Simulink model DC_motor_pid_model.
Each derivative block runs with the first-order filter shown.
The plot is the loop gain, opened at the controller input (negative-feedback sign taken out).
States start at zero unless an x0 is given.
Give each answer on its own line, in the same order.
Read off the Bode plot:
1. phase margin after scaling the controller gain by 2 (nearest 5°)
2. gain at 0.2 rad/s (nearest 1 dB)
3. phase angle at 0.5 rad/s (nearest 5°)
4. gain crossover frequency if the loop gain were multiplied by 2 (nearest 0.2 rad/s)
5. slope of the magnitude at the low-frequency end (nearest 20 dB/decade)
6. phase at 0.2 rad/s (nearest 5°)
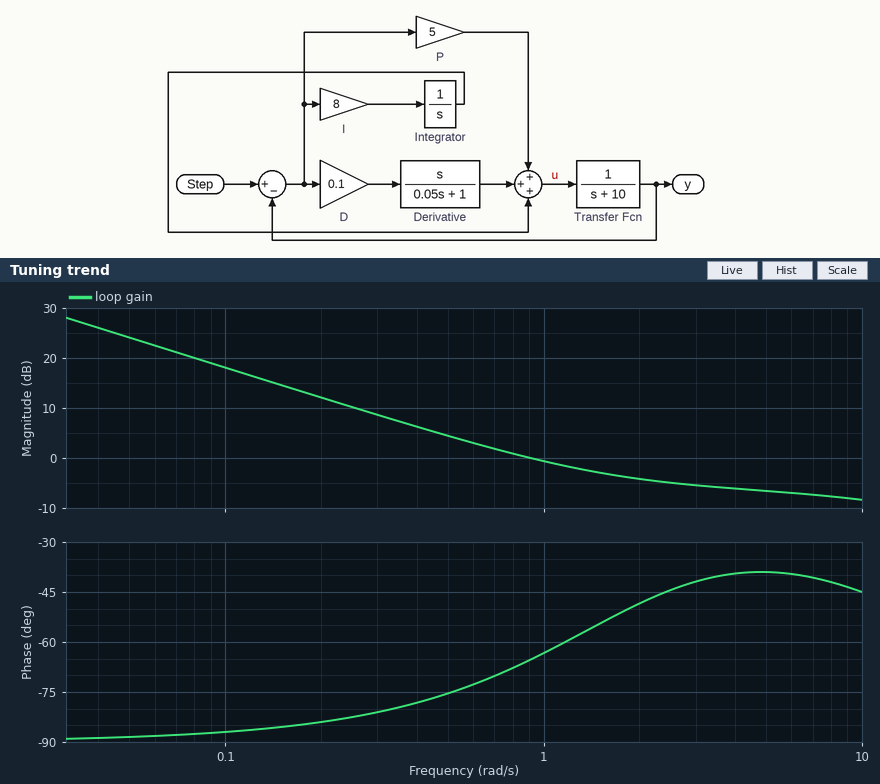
140°
12 dB
-75°
3.8 rad/s
-20 dB/decade
-85°
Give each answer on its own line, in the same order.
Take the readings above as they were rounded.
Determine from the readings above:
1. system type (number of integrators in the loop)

1
